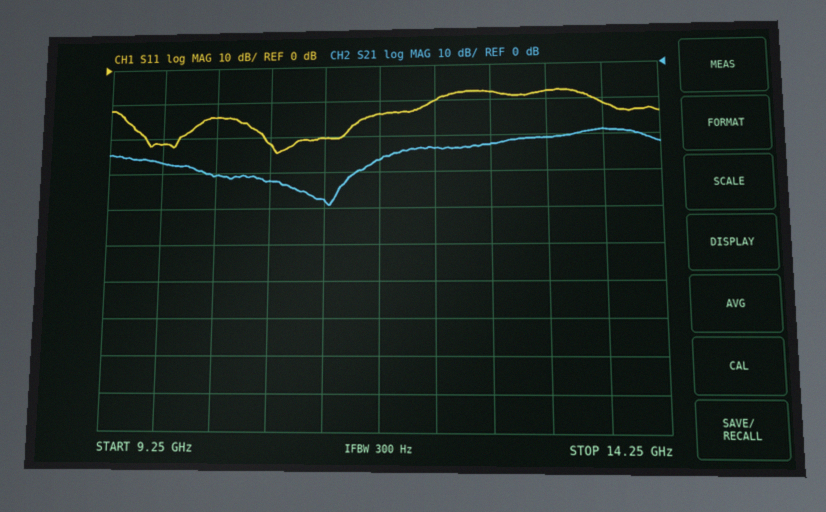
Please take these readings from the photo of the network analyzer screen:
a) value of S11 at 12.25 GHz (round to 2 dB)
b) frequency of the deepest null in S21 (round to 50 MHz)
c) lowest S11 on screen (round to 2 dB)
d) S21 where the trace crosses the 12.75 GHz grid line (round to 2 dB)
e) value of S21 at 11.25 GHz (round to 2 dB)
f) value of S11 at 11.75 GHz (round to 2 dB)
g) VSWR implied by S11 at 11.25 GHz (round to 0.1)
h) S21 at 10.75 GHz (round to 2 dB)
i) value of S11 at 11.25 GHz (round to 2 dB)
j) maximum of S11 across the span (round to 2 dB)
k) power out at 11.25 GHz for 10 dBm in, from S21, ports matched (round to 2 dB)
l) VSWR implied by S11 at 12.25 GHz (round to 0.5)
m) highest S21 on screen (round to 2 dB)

-10 dB
11.30 GHz
-24 dB
-22 dB
-38 dB
-14 dB
1.2
-32 dB
-20 dB
-8 dB
-28 dBm
2.0
-18 dB
